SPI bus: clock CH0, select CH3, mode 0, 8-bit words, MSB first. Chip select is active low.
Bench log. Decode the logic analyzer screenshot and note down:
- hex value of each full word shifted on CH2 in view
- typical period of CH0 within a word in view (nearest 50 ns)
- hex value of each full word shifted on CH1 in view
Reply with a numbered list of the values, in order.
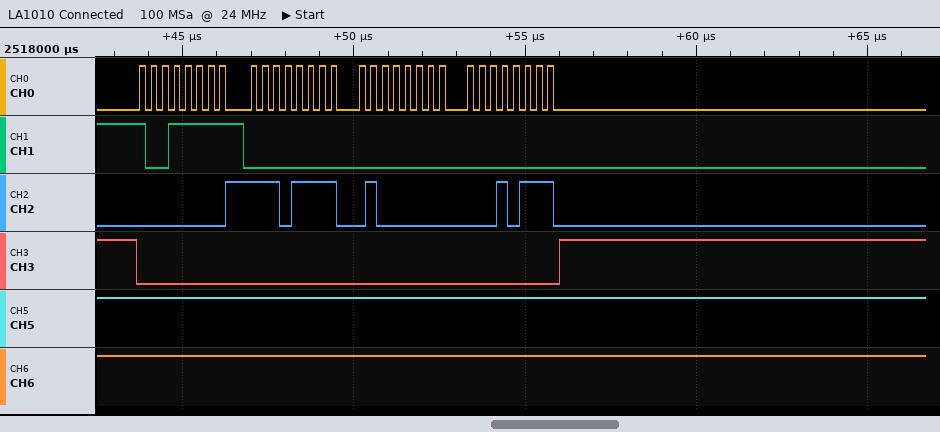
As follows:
1. 00, EF, 40, 17
2. 350 ns
3. 9F, 00, 00, 00
